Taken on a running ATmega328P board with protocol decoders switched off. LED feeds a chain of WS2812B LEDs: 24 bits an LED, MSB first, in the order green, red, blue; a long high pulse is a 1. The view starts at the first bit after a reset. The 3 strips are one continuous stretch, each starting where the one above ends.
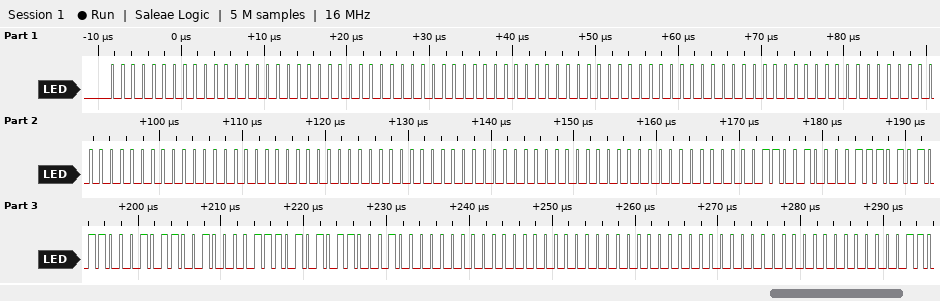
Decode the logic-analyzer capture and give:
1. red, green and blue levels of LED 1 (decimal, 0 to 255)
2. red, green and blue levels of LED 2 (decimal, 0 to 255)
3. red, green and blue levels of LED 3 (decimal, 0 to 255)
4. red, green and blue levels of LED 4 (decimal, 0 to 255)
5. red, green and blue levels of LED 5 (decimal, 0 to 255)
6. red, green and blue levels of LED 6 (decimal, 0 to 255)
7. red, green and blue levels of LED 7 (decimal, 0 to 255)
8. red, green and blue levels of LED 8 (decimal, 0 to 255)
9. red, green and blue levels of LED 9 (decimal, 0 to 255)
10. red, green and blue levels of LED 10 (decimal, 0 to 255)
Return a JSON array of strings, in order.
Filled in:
["0, 0, 0", "0, 0, 0", "0, 0, 0", "0, 0, 0", "0, 0, 0", "0, 0, 0", "58, 100, 177", "58, 100, 177", "0, 0, 0", "0, 0, 0"]
